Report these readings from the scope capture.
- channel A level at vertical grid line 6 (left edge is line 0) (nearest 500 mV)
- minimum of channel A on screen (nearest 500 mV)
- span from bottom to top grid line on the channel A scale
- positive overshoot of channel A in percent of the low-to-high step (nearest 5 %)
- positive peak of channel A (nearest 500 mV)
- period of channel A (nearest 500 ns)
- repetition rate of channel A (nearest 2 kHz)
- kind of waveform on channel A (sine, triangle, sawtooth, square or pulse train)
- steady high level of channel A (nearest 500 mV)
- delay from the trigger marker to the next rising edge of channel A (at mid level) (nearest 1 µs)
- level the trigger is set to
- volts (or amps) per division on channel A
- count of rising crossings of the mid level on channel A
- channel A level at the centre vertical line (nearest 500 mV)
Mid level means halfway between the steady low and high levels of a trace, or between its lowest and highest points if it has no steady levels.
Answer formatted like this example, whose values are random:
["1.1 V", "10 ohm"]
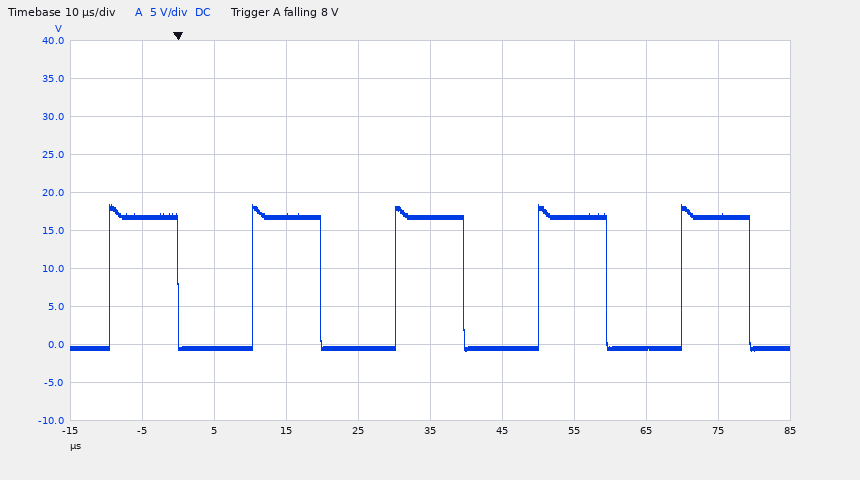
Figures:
["-500 mV", "-1.0 V", "50 V", "10 %", "18.5 V", "20.0 µs", "50 kHz", "square", "17.0 V", "10 µs", "8 V", "5 V", "5", "17.0 V"]
